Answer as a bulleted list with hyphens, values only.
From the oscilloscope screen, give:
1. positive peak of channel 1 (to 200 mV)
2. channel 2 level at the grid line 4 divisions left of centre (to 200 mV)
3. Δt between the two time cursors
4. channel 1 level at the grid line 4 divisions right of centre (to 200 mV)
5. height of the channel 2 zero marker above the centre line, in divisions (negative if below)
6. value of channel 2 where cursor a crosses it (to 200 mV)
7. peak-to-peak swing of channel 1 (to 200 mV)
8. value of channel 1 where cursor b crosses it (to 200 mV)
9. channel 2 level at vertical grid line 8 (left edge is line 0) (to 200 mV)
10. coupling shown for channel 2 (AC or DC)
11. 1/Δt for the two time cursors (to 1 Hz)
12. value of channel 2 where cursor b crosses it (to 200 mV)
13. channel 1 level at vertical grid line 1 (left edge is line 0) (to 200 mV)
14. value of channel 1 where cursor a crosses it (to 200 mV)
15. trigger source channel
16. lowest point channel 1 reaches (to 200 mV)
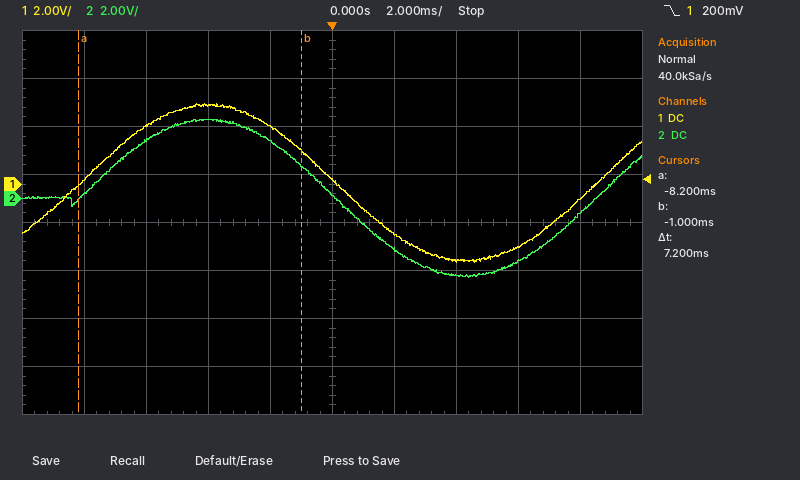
- 3.4 V
- 200 mV
- 7.2 ms
- -600 mV
- +0.5 div
- 0.0 V
- 6.6 V
- 1.4 V
- -2.6 V
- DC
- 139 Hz
- 1.4 V
- 200 mV
- 0.0 V
- channel 1
- -3.2 V
